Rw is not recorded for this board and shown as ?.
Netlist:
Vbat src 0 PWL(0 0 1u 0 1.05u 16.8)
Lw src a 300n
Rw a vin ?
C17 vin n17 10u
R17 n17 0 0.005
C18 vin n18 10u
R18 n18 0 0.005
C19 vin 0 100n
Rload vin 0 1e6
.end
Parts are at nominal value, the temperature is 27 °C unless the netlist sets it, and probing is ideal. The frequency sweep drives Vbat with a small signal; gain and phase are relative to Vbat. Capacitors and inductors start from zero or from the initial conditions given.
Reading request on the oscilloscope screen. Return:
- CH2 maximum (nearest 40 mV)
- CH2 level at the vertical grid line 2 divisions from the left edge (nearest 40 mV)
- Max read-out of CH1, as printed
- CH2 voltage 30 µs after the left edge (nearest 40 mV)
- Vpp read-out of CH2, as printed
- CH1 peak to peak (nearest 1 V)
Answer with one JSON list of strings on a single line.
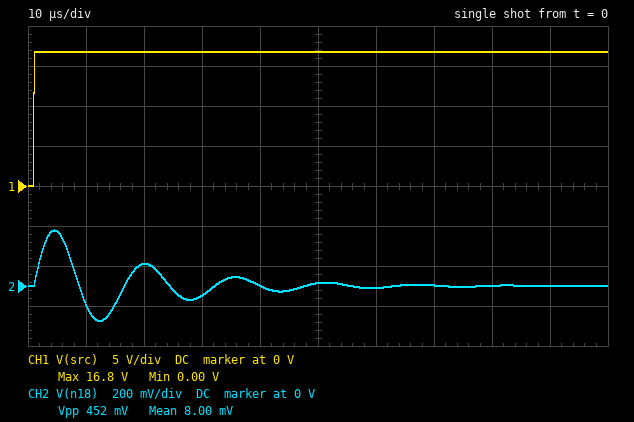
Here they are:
["280 mV", "120 mV", "16.8 V", "-40 mV", "452 mV", "17 V"]
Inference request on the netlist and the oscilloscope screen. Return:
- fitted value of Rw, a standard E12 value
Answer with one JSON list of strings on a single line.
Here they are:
["0.033 Ω"]
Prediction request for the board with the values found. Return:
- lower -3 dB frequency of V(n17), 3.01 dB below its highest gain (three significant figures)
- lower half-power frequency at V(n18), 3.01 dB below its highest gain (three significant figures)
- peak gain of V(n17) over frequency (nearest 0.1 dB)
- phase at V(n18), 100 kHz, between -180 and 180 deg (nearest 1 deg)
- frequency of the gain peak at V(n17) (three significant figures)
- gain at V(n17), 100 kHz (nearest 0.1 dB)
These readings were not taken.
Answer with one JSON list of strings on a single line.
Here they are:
["56.1 kHz", "56.1 kHz", "-23.1 dB", "-72 deg", "64.8 kHz", "-33.3 dB"]
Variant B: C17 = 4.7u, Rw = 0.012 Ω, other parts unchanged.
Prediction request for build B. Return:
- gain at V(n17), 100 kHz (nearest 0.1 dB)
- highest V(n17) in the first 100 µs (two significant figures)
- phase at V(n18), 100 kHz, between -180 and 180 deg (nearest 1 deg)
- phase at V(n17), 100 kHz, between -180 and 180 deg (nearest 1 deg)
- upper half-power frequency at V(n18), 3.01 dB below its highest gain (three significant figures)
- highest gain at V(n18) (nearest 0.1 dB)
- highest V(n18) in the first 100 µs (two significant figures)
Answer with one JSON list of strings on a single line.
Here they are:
["-34.3 dB", "170 mV", "-80 deg", "-79 deg", "79.6 kHz", "-12.8 dB", "370 mV"]
